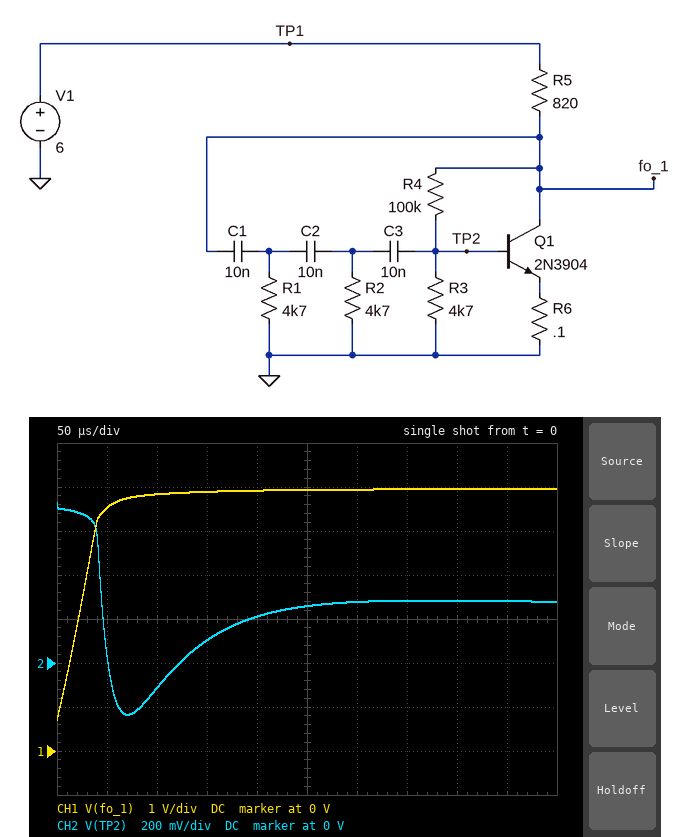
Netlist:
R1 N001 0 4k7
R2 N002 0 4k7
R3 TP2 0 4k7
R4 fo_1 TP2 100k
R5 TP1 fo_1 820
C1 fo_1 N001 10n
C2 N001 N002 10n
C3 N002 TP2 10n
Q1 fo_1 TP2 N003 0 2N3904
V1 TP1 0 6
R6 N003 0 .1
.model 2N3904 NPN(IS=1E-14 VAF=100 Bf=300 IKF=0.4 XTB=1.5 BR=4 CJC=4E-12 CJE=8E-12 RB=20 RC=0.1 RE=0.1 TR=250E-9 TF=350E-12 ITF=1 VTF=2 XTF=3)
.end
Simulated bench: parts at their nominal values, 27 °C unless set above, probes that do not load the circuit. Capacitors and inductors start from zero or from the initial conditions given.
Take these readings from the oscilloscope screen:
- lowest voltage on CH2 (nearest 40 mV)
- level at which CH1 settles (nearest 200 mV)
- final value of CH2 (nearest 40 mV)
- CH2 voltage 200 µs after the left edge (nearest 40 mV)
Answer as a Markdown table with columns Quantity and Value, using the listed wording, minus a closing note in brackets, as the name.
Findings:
| Quantity | Value |
|---|---|
| lowest voltage on CH2 | -240 mV |
| level at which CH1 settles | 6.0 V |
| final value of CH2 | 280 mV |
| CH2 voltage 200 µs after the left edge | 200 mV |
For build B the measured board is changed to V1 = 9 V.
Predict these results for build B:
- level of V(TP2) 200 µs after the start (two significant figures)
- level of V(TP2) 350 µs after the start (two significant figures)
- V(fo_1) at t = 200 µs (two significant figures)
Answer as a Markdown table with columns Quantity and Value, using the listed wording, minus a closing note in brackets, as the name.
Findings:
| Quantity | Value |
|---|---|
| level of V(TP2) 200 µs after the start | 290 mV |
| level of V(TP2) 350 µs after the start | 420 mV |
| V(fo_1) at t = 200 µs | 8.9 V |
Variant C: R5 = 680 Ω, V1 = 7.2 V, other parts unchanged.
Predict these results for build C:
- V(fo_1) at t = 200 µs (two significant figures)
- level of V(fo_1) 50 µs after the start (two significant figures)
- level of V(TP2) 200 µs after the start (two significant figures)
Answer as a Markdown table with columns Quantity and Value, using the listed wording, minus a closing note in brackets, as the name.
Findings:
| Quantity | Value |
|---|---|
| V(fo_1) at t = 200 µs | 7.1 V |
| level of V(fo_1) 50 µs after the start | 6.6 V |
| level of V(TP2) 200 µs after the start | 250 mV |
